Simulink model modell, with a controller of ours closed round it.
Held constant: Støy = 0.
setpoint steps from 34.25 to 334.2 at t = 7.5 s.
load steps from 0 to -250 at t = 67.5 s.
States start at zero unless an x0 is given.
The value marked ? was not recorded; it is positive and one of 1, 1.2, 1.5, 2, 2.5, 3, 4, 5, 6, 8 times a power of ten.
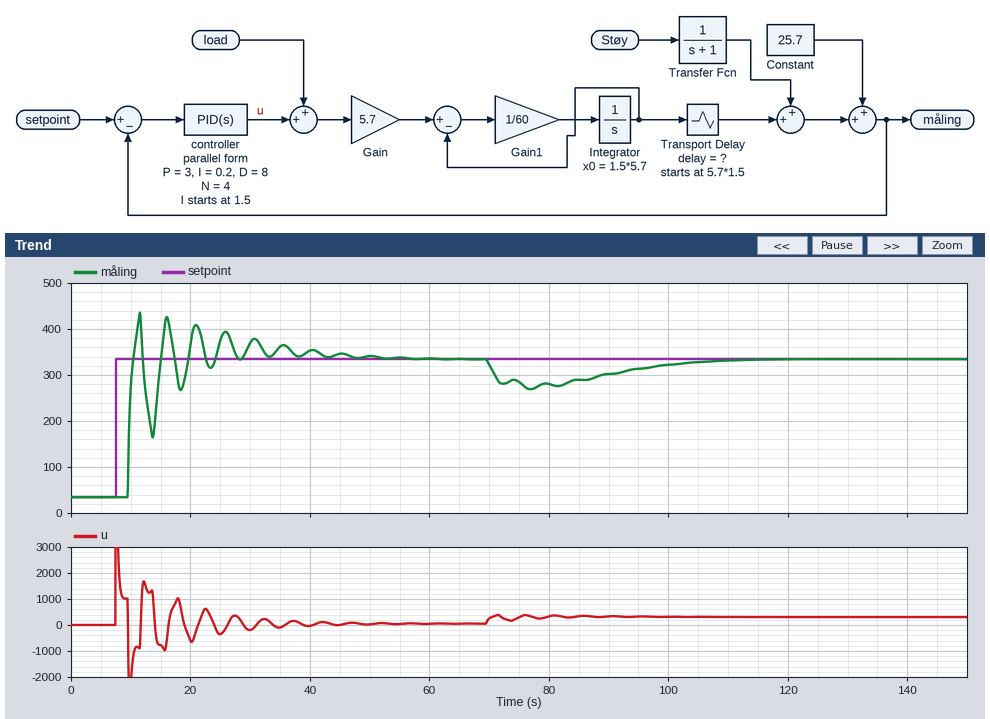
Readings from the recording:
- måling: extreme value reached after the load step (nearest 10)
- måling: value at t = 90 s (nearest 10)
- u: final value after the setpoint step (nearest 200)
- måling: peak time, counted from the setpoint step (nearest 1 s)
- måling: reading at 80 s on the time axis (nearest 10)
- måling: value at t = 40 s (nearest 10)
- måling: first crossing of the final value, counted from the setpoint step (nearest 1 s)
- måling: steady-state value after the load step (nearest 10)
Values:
270
300
0
4 s
280
350
3 s
330
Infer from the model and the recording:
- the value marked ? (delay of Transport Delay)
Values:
2
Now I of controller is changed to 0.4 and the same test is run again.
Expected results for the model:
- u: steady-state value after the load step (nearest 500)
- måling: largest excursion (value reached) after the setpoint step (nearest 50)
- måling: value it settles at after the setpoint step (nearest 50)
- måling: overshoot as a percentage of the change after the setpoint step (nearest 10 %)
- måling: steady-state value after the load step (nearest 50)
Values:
500
450
350
40 %
350
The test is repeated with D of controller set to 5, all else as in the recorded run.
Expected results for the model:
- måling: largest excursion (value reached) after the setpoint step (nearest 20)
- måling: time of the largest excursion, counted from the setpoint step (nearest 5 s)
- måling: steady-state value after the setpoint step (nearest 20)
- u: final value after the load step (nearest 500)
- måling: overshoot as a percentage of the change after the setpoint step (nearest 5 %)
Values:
360
15 s
340
500
10 %
